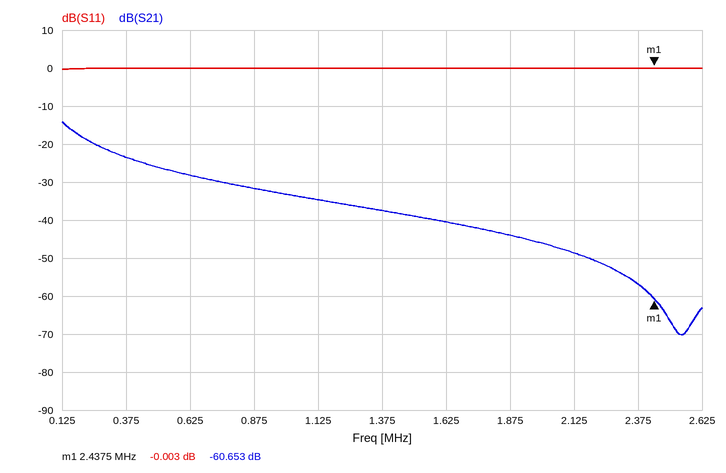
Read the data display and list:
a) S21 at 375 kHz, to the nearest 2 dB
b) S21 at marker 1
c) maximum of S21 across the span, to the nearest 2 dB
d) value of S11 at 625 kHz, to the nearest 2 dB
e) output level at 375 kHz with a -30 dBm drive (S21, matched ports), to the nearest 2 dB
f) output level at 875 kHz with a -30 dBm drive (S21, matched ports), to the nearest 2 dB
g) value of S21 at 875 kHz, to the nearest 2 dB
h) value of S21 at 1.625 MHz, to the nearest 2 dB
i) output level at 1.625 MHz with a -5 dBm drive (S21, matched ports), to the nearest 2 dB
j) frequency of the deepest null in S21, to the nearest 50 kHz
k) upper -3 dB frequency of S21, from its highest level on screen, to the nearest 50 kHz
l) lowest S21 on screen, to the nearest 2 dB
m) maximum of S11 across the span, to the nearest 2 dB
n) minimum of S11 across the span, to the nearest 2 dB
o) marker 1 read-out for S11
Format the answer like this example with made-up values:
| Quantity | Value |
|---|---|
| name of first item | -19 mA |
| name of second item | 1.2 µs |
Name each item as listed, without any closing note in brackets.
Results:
| Quantity | Value |
|---|---|
| S21 at 375 kHz, to the nearest 2 dB | -24 dB |
| S21 at marker 1 | -60.653 dB |
| maximum of S21 across the span, to the nearest 2 dB | -14 dB |
| value of S11 at 625 kHz, to the nearest 2 dB | 0 dB |
| output level at 375 kHz with a -30 dBm drive (S21, matched ports), to the nearest 2 dB | -54 dBm |
| output level at 875 kHz with a -30 dBm drive (S21, matched ports), to the nearest 2 dB | -62 dBm |
| value of S21 at 875 kHz, to the nearest 2 dB | -32 dB |
| value of S21 at 1.625 MHz, to the nearest 2 dB | -40 dB |
| output level at 1.625 MHz with a -5 dBm drive (S21, matched ports), to the nearest 2 dB | -46 dBm |
| frequency of the deepest null in S21, to the nearest 50 kHz | 2.55 MHz |
| upper -3 dB frequency of S21, from its highest level on screen, to the nearest 50 kHz | 200 kHz |
| lowest S21 on screen, to the nearest 2 dB | -70 dB |
| maximum of S11 across the span, to the nearest 2 dB | 0 dB |
| minimum of S11 across the span, to the nearest 2 dB | 0 dB |
| marker 1 read-out for S11 | -0.003 dB |
